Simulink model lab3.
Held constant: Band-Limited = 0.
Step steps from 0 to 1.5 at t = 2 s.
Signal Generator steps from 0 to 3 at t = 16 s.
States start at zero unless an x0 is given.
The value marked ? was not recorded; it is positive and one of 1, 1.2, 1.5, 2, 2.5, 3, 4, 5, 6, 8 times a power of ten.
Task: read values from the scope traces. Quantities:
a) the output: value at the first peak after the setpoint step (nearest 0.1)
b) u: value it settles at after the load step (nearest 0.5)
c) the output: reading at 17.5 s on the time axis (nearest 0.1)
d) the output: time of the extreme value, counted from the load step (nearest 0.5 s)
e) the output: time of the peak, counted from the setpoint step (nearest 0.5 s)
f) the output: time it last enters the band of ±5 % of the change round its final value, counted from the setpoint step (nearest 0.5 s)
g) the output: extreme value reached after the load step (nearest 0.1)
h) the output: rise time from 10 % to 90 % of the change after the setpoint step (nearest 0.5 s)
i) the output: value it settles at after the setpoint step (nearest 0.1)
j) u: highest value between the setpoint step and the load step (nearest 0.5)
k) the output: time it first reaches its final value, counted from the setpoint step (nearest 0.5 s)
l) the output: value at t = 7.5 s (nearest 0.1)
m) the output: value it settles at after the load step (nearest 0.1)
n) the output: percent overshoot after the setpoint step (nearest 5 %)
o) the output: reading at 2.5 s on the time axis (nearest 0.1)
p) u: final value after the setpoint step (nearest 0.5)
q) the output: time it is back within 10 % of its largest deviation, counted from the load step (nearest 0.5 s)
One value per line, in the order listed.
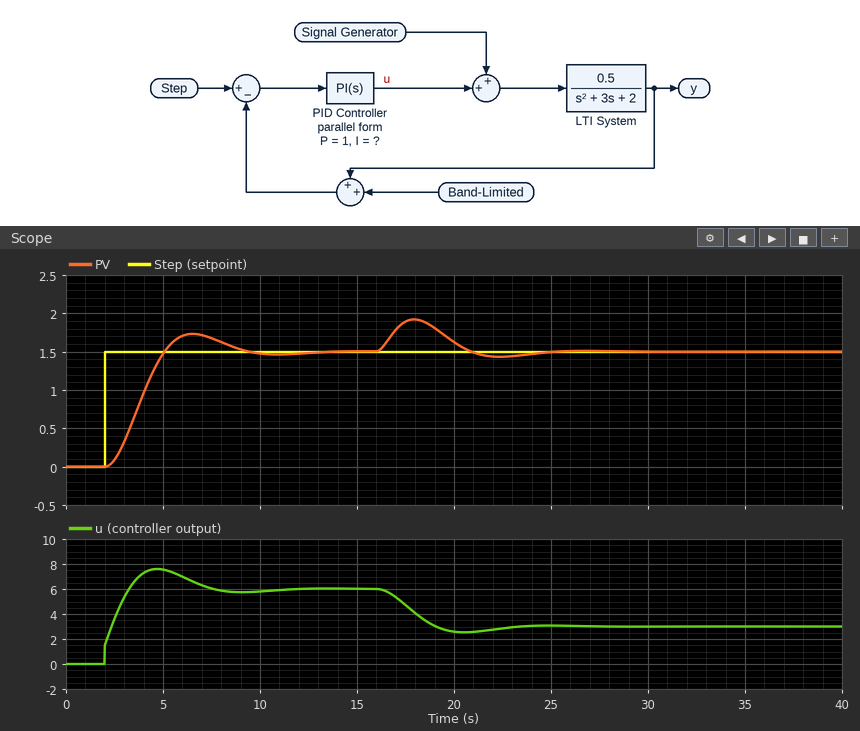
1.7
3.0
1.9
2.0 s
4.5 s
6.5 s
1.9
2.0 s
1.5
7.5
3.0 s
1.7
1.5
15 %
0.1
6.0
7.5 s
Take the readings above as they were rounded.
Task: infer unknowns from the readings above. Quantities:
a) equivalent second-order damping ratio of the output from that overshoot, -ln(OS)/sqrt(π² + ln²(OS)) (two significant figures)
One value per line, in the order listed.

0.52
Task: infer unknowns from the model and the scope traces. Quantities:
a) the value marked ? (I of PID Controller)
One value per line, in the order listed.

3
